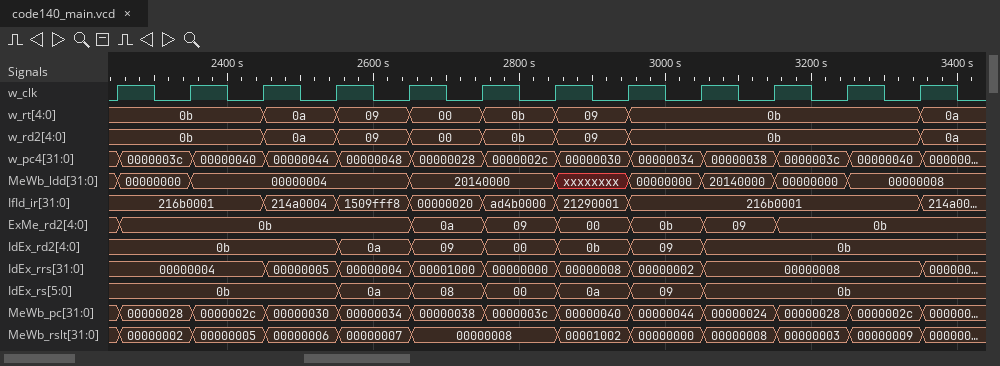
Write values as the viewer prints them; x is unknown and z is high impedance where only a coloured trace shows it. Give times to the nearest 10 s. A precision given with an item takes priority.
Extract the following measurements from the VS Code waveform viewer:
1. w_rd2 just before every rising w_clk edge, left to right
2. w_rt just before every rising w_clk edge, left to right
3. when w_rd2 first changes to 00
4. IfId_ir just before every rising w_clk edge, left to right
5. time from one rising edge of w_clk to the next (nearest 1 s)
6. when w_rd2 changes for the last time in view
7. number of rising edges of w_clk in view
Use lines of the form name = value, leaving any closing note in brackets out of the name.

w_rd2 just before every rising w_clk edge, left to right = 0b, 0b, 0b, 0a, 09, 00, 0b, 09, 0b, 0b, 0b, 0b
w_rt just before every rising w_clk edge, left to right = 0b, 0b, 0b, 0a, 09, 00, 0b, 09, 0b, 0b, 0b, 0b
when w_rd2 first changes to 00 = 2650 s
IfId_ir just before every rising w_clk edge, left to right = 216b0001, 216b0001, 216b0001, 214a0004, 1509fff8, 00000020, ad4b0000, 21290001, 216b0001, 216b0001, 216b0001, 216b0001
time from one rising edge of w_clk to the next = 100 s
when w_rd2 changes for the last time in view = 3350 s
number of rising edges of w_clk in view = 12
